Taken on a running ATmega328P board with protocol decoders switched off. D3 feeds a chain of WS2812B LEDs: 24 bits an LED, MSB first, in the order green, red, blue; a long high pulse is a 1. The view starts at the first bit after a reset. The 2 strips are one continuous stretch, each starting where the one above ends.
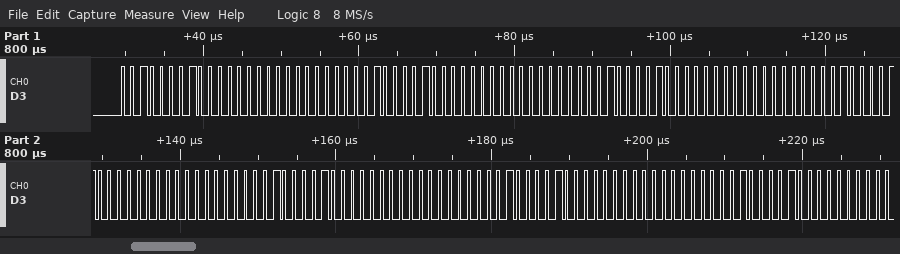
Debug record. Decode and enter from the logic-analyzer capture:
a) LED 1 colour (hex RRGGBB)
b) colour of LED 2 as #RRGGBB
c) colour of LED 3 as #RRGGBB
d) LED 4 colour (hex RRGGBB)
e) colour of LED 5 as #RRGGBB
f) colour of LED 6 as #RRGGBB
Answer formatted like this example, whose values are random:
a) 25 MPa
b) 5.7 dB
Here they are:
a) #002100
b) #002100
c) #002100
d) #002100
e) #002100
f) #002100
